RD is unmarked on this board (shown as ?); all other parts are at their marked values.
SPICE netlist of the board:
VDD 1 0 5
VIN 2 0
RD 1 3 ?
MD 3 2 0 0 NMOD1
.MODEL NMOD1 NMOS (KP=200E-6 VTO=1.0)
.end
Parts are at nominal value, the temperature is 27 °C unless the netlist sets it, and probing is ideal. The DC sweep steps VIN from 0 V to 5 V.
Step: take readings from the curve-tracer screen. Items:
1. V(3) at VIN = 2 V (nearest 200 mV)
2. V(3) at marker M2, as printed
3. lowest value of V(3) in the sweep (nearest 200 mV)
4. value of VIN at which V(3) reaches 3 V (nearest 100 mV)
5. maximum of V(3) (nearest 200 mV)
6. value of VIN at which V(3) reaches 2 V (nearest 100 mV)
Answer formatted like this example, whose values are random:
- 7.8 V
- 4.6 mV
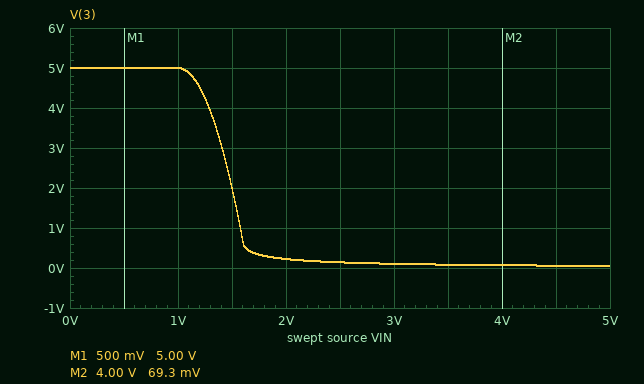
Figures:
- 200 mV
- 69.3 mV
- 0 V
- 1.4 V
- 5.0 V
- 1.5 V
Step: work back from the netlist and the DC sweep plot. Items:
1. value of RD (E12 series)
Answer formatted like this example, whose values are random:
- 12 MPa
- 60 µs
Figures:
- 120 kΩ
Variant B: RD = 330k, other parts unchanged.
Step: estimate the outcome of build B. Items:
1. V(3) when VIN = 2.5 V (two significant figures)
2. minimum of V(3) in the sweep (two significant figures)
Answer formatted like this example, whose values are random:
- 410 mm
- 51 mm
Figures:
- 51 mV
- 19 mV
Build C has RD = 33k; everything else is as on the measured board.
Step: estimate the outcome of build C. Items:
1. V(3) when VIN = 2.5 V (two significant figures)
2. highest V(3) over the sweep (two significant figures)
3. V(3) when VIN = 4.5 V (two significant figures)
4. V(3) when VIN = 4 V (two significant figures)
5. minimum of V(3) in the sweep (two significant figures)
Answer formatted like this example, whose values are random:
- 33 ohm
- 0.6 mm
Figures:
- 550 mV
- 5.0 V
- 210 mV
- 250 mV
- 190 mV
